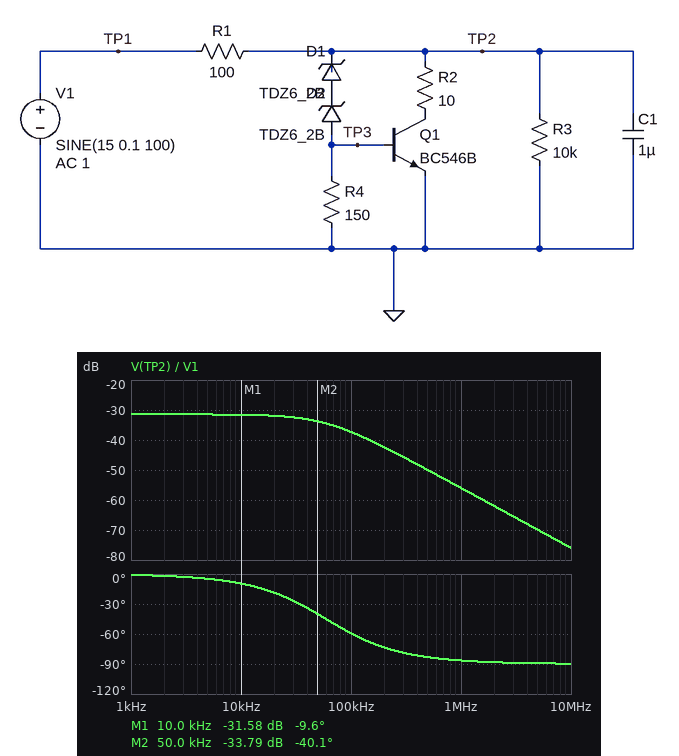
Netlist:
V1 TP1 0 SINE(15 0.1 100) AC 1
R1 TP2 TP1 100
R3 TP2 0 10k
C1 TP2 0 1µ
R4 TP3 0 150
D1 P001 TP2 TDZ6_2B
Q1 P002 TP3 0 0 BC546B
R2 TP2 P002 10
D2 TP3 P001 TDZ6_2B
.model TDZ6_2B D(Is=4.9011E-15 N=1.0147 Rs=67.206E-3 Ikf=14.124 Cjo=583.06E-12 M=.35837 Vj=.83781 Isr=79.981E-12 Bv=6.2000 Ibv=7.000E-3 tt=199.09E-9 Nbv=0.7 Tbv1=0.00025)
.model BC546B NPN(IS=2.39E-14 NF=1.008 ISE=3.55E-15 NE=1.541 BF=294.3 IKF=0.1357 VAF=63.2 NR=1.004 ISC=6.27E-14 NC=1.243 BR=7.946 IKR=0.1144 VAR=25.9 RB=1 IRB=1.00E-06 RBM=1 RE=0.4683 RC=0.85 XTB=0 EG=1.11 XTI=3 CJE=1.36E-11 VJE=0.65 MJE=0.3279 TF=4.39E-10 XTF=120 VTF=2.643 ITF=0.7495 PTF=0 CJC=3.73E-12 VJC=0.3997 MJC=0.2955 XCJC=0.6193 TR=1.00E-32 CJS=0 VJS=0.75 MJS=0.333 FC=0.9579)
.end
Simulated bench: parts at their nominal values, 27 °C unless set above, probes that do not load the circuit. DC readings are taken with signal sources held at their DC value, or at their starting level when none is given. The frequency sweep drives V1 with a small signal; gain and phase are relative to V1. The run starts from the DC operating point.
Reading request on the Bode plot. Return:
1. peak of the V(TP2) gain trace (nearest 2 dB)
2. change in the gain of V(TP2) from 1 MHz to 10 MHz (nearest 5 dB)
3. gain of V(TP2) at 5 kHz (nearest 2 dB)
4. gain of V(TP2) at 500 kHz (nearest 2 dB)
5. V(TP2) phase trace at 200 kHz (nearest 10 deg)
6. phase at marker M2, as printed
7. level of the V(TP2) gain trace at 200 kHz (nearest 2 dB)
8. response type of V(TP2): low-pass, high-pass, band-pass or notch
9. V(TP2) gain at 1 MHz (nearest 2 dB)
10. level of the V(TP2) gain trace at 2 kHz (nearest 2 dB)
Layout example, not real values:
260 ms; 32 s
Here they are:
-32 dB; -20 dB; -32 dB; -50 dB; -70 deg; -40.1 deg; -42 dB; low-pass; -56 dB; -32 dB
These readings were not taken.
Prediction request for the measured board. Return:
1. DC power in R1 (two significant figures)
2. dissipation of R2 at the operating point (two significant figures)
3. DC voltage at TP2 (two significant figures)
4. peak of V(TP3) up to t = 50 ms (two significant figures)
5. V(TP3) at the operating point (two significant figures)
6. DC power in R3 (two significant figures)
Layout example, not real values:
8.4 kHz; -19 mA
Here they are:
36 mW; 1.7 mW; 13 V; 710 mV; 710 mV; 17 mW
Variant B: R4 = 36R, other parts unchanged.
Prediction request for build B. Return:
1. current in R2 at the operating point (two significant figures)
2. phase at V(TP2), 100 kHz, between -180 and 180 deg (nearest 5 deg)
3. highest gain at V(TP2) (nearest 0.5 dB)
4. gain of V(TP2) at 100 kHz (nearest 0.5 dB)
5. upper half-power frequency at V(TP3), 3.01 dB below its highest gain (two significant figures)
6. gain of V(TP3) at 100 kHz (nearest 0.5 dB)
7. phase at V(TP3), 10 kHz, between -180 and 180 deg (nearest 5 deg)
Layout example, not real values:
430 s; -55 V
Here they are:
720 µA; -85 deg; -16.0 dB; -36.0 dB; 9.8 kHz; -36.5 dB; -45 deg
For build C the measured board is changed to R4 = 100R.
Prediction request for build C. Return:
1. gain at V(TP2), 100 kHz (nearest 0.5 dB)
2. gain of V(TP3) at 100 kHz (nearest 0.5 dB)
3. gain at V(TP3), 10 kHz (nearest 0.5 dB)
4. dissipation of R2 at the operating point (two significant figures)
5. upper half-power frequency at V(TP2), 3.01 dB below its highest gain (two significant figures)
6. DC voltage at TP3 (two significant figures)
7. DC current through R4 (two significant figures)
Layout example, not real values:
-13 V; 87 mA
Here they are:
-37.0 dB; -37.5 dB; -31.0 dB; 1.1 mW; 52 kHz; 700 mV; 7.0 mA
